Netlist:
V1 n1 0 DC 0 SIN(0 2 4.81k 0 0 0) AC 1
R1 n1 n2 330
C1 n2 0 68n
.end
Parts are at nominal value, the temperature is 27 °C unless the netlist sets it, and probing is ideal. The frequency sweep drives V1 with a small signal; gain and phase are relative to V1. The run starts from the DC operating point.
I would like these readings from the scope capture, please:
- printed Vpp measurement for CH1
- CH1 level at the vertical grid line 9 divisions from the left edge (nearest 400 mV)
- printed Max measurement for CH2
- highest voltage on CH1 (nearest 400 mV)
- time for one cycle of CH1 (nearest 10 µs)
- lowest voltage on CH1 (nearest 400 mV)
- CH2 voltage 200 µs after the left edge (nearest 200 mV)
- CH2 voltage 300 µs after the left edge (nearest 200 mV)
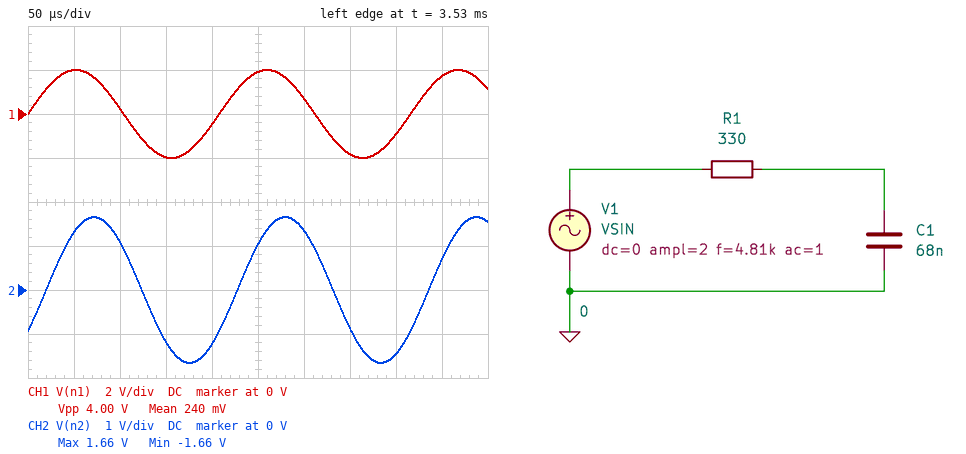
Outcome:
4.00 V
1.6 V
1.66 V
2.0 V
210 µs
-2.0 V
-1.2 V
1.4 V
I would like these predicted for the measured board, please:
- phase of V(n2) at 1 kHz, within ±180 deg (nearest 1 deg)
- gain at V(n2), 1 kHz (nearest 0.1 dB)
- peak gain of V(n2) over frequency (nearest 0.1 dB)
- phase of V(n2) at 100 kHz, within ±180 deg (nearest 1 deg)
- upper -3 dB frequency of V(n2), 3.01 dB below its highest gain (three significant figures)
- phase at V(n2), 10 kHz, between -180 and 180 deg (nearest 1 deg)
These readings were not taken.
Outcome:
-8 deg
-0.1 dB
0 dB
-86 deg
7.09 kHz
-55 deg
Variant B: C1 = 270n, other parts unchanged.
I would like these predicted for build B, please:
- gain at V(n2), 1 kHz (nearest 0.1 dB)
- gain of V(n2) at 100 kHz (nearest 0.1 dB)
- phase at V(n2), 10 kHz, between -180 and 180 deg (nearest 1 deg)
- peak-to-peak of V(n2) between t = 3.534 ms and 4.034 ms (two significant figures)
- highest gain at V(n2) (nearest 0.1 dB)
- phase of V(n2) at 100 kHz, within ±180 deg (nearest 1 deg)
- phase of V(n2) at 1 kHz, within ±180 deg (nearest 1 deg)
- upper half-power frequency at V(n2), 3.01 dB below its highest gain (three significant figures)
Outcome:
-1.2 dB
-35.0 dB
-80 deg
1.4 V
0 dB
-89 deg
-29 deg
1.79 kHz
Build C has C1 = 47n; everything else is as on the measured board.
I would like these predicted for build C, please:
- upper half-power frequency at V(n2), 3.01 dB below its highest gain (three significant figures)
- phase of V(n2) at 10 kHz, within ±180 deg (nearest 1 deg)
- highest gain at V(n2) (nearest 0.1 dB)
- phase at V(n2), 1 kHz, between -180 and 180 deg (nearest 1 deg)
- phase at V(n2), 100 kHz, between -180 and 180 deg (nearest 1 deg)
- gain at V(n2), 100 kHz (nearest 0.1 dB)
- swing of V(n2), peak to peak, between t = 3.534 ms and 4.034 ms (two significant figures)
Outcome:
10.3 kHz
-44 deg
0 dB
-6 deg
-84 deg
-19.8 dB
3.6 V
